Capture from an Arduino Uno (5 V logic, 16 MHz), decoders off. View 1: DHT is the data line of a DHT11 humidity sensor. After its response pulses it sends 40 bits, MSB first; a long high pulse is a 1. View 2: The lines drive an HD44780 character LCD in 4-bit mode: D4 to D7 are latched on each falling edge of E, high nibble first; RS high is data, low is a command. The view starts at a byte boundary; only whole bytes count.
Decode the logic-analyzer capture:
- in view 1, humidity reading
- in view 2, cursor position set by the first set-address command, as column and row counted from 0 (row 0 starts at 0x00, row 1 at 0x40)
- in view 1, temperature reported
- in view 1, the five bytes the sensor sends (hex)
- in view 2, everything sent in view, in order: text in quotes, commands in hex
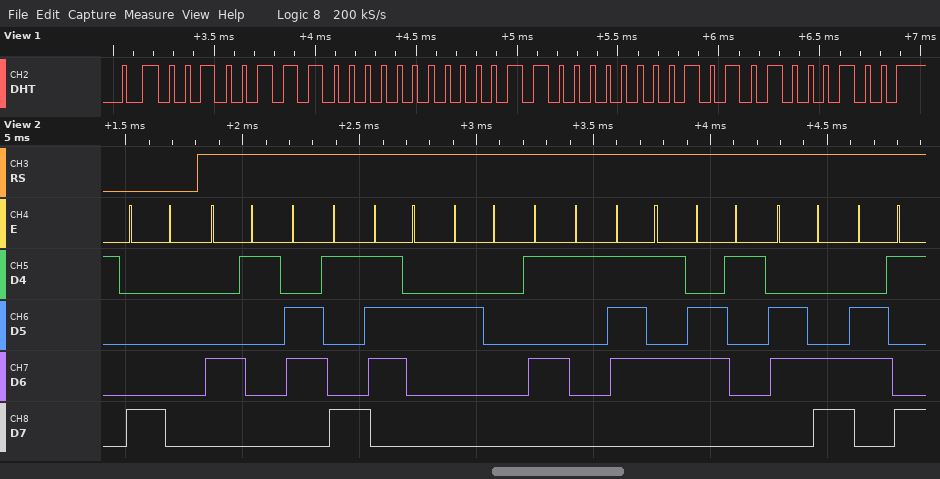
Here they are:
39 %
column 0, row 0
24.5 °C
27 00 18 05 44
0x80 "Air Quali"
